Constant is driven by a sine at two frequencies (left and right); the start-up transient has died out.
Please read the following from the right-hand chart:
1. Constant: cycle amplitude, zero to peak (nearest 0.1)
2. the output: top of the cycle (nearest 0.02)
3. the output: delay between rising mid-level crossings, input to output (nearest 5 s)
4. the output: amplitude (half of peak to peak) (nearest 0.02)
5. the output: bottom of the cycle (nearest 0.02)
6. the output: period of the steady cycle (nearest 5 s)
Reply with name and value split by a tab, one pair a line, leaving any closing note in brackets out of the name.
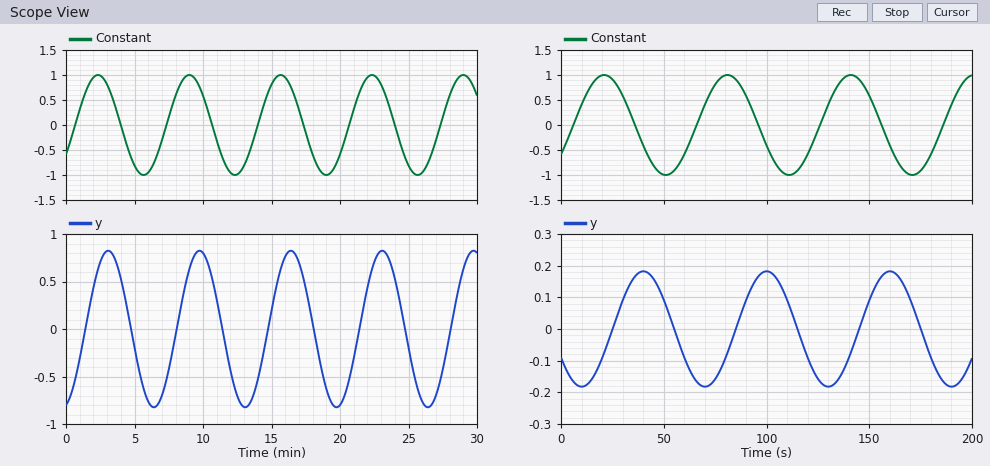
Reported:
Constant: cycle amplitude, zero to peak	1.0
the output: top of the cycle	0.18
the output: delay between rising mid-level crossings, input to output	20 s
the output: amplitude (half of peak to peak)	0.18
the output: bottom of the cycle	-0.18
the output: period of the steady cycle	60 s
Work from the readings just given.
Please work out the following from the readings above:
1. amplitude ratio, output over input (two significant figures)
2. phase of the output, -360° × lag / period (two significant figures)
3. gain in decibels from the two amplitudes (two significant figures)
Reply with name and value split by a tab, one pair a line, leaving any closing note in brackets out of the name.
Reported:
amplitude ratio, output over input	0.18
phase of the output, -360° × lag / period	-120°
gain in decibels from the two amplitudes	-15 dB
